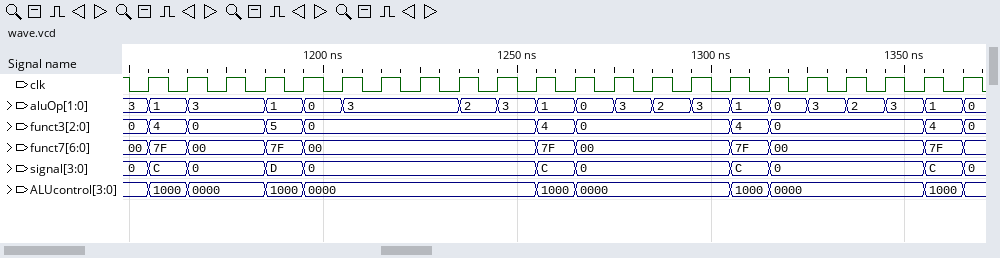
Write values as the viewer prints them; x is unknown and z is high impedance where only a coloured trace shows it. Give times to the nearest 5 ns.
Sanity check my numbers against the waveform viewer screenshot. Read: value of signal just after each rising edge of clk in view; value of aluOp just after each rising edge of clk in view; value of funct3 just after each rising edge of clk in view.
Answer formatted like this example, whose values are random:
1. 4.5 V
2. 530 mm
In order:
1. C, 0, 0, D, 0, 0, 0, 0, 0, 0, C, 0, 0, 0, 0, C, 0, 0, 0, 0, C, 0
2. 1, 3, 3, 1, 0, 3, 3, 3, 2, 3, 1, 0, 3, 2, 3, 1, 0, 3, 2, 3, 1, 0
3. 4, 0, 0, 5, 0, 0, 0, 0, 0, 0, 4, 0, 0, 0, 0, 4, 0, 0, 0, 0, 4, 0
